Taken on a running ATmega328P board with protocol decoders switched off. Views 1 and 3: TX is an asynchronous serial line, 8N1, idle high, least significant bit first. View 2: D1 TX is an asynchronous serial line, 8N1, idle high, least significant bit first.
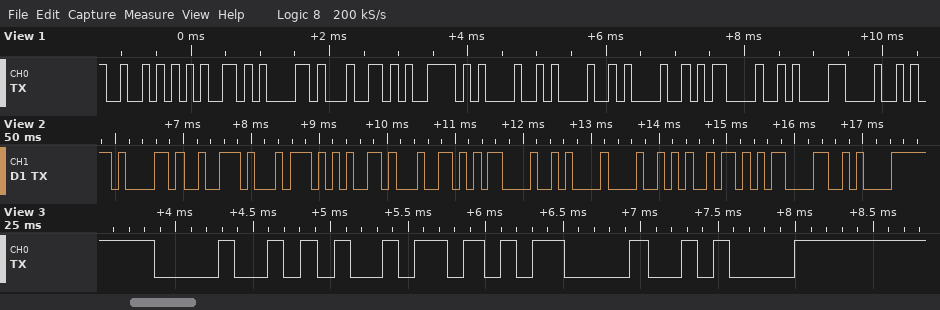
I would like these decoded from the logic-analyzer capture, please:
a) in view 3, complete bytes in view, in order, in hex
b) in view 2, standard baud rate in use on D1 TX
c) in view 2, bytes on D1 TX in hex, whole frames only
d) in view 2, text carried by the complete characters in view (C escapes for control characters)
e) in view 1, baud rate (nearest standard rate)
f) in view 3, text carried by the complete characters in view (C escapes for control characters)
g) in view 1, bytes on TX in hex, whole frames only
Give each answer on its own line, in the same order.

48 69 0D 0A
9600 baud
61 72 74 65 64 0D 0A 48 69 0D 0A
"arted\r\nHi\r\n"
9600 baud
"Hi\r\n"
0x52 0x65 0x61 0x64 0x79 0x21 0x21 0x21 0x0D 0x0A 0x48
